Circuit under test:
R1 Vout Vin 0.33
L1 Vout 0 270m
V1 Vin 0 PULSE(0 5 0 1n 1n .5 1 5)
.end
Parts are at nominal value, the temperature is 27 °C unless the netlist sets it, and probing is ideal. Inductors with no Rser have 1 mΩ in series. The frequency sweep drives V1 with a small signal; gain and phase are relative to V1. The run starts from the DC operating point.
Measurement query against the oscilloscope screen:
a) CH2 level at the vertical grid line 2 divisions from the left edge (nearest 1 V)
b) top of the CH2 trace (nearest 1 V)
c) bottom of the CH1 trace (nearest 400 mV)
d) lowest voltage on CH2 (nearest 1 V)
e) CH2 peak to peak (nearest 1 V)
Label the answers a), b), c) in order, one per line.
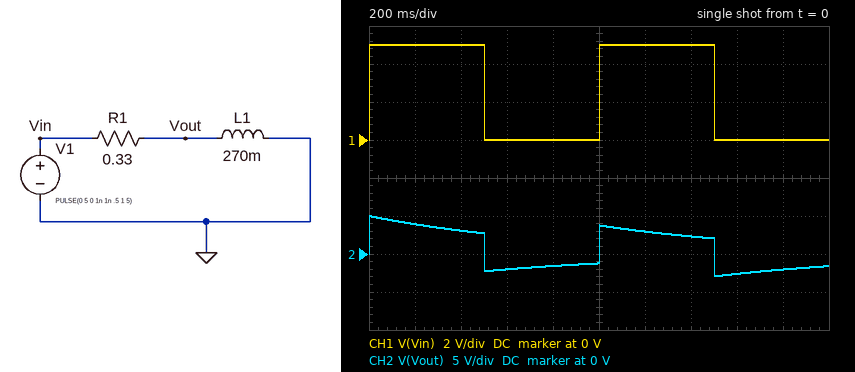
a) 3 V
b) 5 V
c) 0 V
d) -3 V
e) 8 V
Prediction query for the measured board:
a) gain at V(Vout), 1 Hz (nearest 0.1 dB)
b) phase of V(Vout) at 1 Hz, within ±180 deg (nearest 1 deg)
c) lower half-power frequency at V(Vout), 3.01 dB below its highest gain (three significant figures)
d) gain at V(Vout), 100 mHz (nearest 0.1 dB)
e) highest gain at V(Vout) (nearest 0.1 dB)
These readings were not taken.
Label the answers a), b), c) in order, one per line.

a) -0.2 dB
b) 11 deg
c) 195 mHz
d) -6.8 dB
e) 0 dB
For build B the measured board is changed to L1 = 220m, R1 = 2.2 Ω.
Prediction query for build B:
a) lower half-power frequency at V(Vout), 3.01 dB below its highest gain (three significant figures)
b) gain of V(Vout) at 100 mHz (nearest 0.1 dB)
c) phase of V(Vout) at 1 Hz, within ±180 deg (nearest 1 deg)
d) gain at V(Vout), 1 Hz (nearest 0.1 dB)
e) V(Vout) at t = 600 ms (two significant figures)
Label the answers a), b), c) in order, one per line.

a) 1.59 Hz
b) -24.1 dB
c) 58 deg
d) -5.5 dB
e) -1.8 V
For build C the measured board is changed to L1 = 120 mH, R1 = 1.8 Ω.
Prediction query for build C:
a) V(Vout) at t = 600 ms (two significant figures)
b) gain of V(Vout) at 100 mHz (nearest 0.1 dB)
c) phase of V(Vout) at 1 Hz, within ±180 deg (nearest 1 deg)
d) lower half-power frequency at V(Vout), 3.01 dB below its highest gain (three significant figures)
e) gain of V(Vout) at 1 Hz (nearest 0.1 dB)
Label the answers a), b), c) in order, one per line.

a) -1.1 V
b) -27.6 dB
c) 67 deg
d) 2.39 Hz
e) -8.3 dB
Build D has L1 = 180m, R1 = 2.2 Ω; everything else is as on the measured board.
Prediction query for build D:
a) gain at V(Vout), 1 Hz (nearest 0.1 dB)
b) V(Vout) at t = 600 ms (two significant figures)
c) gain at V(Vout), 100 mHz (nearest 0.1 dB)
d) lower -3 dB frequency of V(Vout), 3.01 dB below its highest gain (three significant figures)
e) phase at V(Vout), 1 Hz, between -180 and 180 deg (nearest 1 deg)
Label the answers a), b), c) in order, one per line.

a) -6.8 dB
b) -1.5 V
c) -25.8 dB
d) 1.95 Hz
e) 63 deg
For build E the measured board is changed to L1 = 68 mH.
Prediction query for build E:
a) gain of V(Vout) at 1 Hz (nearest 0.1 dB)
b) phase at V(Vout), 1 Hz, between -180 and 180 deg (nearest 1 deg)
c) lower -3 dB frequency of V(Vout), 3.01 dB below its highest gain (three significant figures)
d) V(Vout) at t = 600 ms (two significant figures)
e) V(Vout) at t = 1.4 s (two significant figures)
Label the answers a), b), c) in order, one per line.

a) -2.0 dB
b) 38 deg
c) 775 mHz
d) -2.8 V
e) 670 mV
